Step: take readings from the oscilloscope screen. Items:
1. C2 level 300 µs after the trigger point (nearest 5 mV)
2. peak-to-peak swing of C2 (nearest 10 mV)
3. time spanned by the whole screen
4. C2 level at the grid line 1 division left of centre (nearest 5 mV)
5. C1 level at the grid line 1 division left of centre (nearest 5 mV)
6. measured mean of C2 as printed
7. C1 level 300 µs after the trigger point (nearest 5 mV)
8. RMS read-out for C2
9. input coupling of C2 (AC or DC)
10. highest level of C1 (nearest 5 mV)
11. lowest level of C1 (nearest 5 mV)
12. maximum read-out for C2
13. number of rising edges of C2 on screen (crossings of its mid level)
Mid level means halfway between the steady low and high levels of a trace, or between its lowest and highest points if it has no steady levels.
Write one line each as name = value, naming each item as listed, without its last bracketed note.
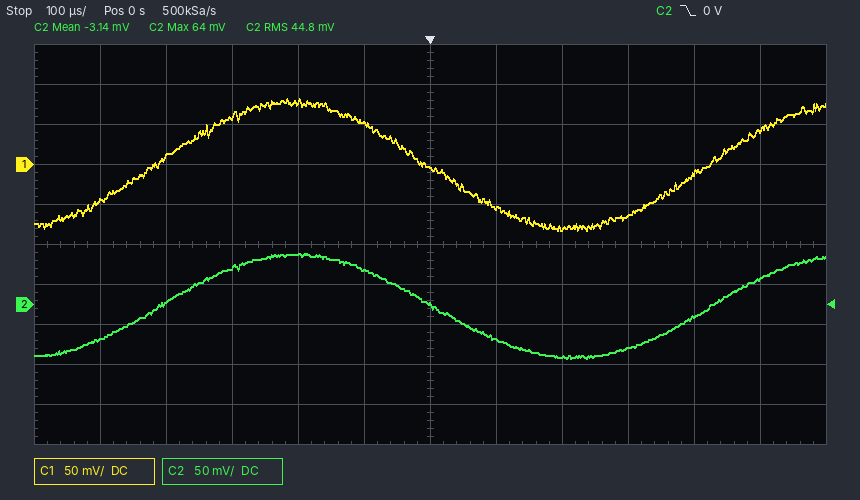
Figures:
C2 level 300 µs after the trigger point = -55 mV
peak-to-peak swing of C2 = 130 mV
time spanned by the whole screen = 1.2 ms
C2 level at the grid line 1 division left of centre = 45 mV
C1 level at the grid line 1 division left of centre = 50 mV
measured mean of C2 as printed = -3.14 mV
C1 level 300 µs after the trigger point = -65 mV
RMS read-out for C2 = 44.8 mV
input coupling of C2 = DC
highest level of C1 = 80 mV
lowest level of C1 = -80 mV
maximum read-out for C2 = 64 mV
number of rising edges of C2 on screen = 2
